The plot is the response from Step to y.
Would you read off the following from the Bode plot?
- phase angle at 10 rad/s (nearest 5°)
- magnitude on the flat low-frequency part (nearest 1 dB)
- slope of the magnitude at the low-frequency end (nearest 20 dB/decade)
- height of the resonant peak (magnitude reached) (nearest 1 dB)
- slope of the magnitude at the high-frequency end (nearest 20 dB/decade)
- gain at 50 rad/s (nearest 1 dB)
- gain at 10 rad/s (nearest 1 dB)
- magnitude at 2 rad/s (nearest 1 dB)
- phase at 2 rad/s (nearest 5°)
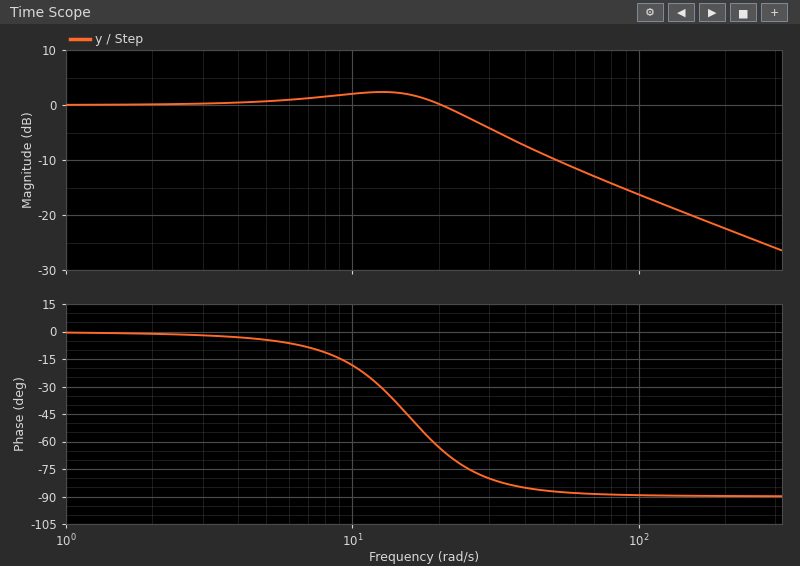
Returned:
-20°
0 dB
0 dB/decade
2 dB
-20 dB/decade
-10 dB
2 dB
0 dB
0°
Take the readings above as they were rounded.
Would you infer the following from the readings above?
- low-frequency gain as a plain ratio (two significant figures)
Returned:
1.0
